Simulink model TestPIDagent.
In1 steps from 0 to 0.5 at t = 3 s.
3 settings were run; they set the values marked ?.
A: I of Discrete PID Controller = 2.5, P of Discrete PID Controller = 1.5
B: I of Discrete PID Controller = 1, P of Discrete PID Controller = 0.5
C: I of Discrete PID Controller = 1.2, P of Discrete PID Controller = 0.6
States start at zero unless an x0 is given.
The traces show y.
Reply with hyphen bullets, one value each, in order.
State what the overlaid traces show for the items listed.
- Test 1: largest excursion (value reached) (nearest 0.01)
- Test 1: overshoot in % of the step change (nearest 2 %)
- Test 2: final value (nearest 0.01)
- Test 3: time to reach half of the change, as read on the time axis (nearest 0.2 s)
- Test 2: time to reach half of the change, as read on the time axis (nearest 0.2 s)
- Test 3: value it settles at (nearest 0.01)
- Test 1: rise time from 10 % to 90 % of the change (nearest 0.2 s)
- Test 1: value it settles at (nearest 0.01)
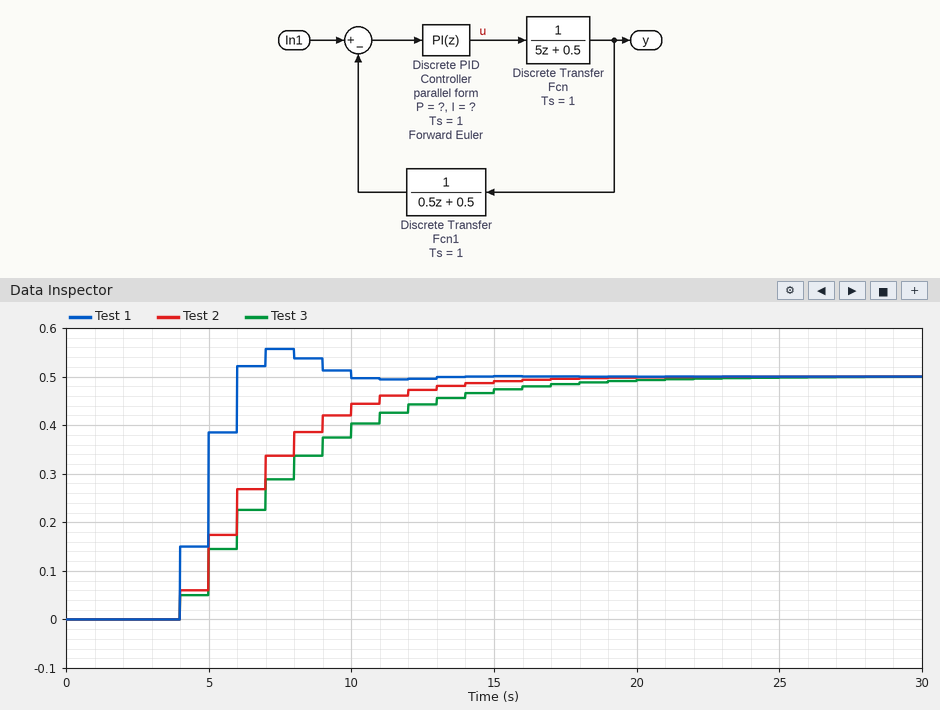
- 0.56
- 12 %
- 0.50
- 7.0 s
- 6.0 s
- 0.50
- 2.0 s
- 0.50
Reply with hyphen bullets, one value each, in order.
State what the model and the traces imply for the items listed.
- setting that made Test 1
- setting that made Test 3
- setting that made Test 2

- A
- B
- C
